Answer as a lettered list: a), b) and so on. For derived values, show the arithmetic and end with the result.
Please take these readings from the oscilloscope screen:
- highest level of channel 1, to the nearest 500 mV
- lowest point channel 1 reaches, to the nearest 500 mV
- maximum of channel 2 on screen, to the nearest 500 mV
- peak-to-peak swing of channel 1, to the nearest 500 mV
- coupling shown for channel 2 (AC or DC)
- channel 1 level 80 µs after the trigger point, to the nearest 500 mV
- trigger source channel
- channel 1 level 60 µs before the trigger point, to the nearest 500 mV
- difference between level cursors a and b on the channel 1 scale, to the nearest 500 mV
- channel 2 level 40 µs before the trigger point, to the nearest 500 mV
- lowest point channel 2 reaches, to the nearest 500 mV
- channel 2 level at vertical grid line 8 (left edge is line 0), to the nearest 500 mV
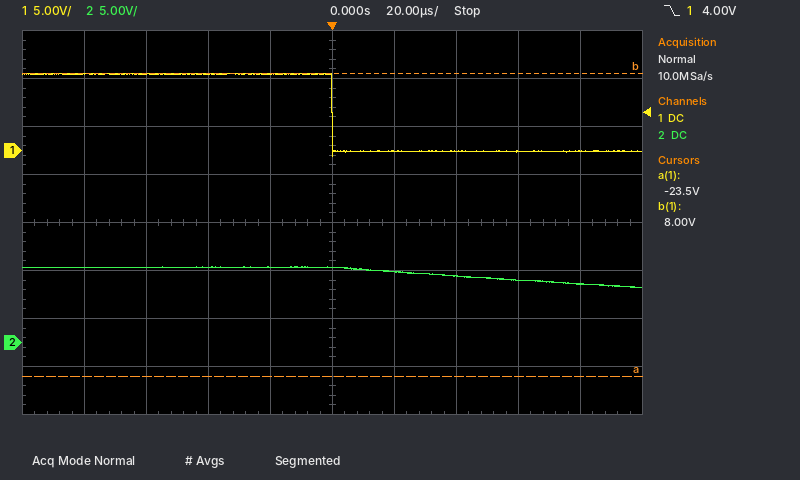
a) 8.0 V
b) -500 mV
c) 8.0 V
d) 8.0 V − (-500 mV) = 8.5 V
e) DC
f) 0.0 V
g) channel 1
h) 8.0 V
i) 31.5 V
j) 8.0 V
k) 5.5 V
l) 6.5 V
